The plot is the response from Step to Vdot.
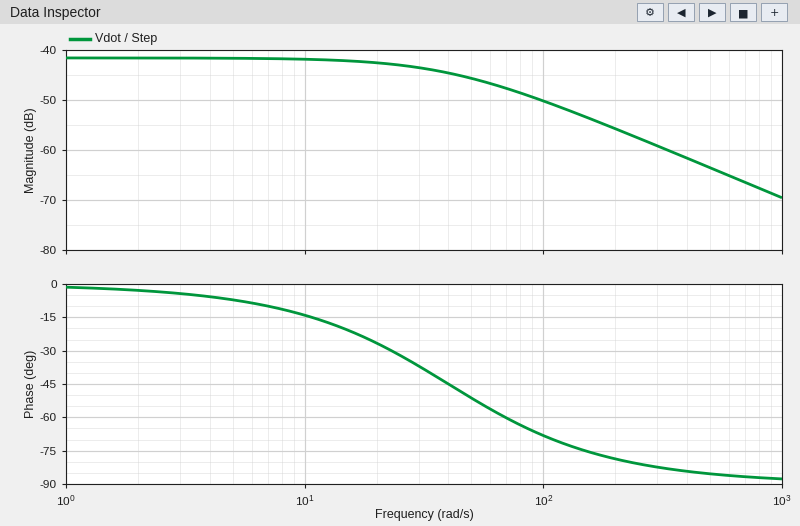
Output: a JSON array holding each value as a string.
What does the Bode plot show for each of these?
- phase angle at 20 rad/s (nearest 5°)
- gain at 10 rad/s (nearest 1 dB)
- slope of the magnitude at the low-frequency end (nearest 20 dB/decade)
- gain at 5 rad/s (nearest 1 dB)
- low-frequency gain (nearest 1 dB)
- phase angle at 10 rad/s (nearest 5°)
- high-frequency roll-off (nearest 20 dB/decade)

["-25°", "-42 dB", "0 dB/decade", "-42 dB", "-42 dB", "-15°", "-20 dB/decade"]
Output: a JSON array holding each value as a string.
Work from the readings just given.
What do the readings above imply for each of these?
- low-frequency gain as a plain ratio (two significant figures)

["0.0079"]
